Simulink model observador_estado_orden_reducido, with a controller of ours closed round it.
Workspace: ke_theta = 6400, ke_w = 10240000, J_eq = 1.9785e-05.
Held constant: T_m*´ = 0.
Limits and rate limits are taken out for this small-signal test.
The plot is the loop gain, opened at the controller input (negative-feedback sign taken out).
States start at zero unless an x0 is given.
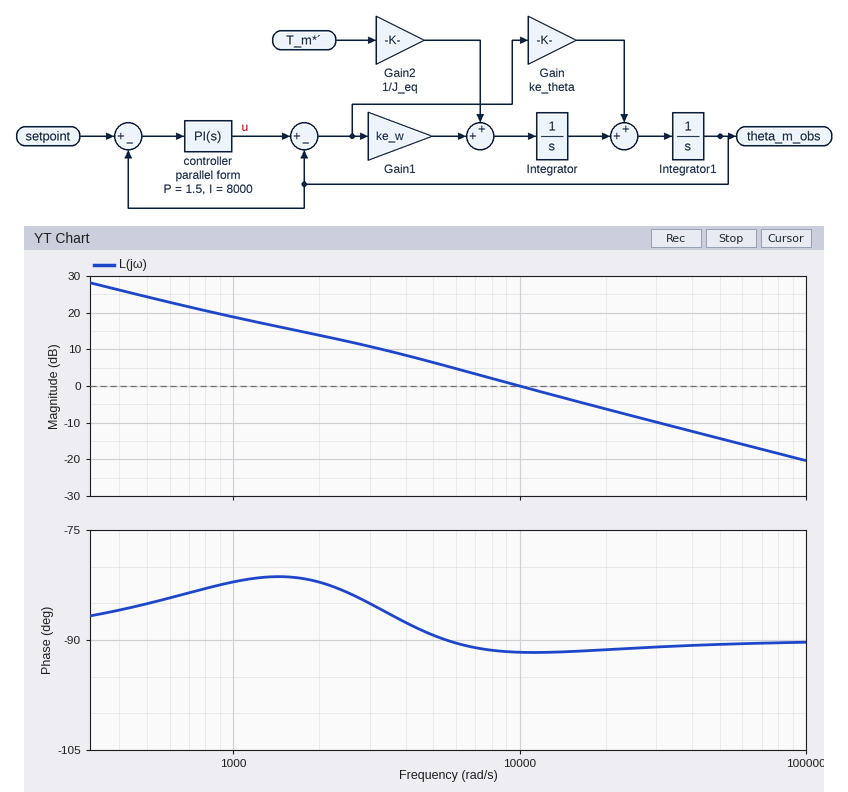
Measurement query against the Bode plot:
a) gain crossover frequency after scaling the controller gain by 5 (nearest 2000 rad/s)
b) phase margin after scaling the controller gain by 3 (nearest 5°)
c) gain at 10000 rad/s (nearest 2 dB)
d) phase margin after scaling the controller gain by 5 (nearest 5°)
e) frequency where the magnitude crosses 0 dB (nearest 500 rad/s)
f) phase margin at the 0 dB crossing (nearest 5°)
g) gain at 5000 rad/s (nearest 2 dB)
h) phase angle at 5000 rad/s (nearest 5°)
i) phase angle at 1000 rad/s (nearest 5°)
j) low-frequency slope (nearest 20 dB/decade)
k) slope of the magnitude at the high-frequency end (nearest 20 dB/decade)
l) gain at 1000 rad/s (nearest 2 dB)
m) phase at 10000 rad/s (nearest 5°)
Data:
48000 rad/s
90°
0 dB
90°
10000 rad/s
90°
6 dB
-90°
-80°
-20 dB/decade
-20 dB/decade
18 dB
-90°
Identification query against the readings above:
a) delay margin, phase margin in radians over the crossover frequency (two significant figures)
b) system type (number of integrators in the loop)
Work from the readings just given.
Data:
0.00016 s
1
